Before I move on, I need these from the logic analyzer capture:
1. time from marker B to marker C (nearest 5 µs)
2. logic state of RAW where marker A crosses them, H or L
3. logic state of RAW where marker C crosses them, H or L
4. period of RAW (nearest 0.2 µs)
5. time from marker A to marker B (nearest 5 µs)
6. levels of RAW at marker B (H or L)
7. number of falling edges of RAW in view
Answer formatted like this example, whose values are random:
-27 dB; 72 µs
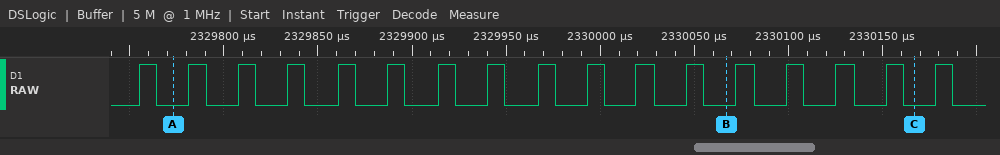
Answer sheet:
100 µs; RAW=L; RAW=L; 26.4 µs; 295 µs; RAW=L; 17
